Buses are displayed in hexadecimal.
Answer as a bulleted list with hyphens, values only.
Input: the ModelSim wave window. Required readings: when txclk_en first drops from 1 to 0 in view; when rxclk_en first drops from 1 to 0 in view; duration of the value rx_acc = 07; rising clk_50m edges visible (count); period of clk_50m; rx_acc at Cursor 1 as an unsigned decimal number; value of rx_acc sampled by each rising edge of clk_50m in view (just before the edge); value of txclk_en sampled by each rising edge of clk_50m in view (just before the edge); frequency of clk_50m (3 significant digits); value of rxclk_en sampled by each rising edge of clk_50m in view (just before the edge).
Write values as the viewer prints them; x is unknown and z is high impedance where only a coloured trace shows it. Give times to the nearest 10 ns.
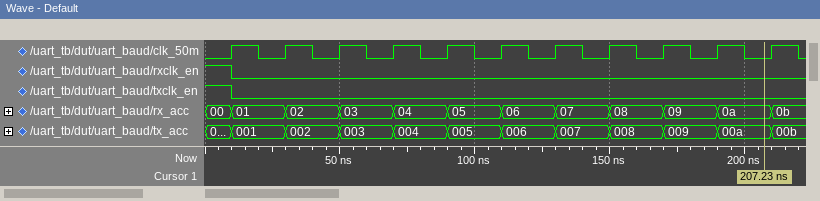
- 10 ns
- 10 ns
- 20 ns
- 11
- 20 ns
- 10
- 00, 01, 02, 03, 04, 05, 06, 07, 08, 09, 0a
- 1 0 0 0 0 0 0 0 0 0 0
- 50.0 MHz
- 1 0 0 0 0 0 0 0 0 0 0
